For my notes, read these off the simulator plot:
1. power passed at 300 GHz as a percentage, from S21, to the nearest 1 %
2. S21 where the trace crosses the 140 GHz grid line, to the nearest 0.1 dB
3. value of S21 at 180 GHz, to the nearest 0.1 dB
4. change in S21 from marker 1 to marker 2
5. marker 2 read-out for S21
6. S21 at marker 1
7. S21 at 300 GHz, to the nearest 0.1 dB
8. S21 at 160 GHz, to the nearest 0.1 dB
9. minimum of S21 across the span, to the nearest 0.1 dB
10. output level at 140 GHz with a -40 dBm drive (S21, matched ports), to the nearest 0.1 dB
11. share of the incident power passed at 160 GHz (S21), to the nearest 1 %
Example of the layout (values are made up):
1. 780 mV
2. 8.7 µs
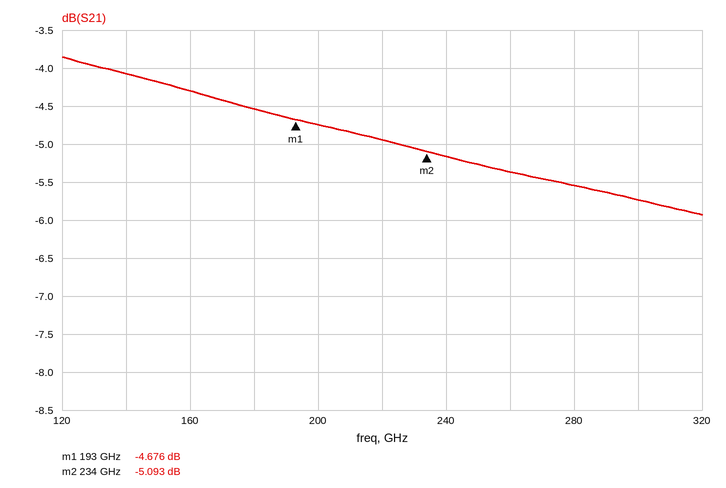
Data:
1. 27 %
2. -4.1 dB
3. -4.5 dB
4. -0.417 dB
5. -5.093 dB
6. -4.676 dB
7. -5.7 dB
8. -4.3 dB
9. -5.9 dB
10. -44.1 dBm
11. 37 %
